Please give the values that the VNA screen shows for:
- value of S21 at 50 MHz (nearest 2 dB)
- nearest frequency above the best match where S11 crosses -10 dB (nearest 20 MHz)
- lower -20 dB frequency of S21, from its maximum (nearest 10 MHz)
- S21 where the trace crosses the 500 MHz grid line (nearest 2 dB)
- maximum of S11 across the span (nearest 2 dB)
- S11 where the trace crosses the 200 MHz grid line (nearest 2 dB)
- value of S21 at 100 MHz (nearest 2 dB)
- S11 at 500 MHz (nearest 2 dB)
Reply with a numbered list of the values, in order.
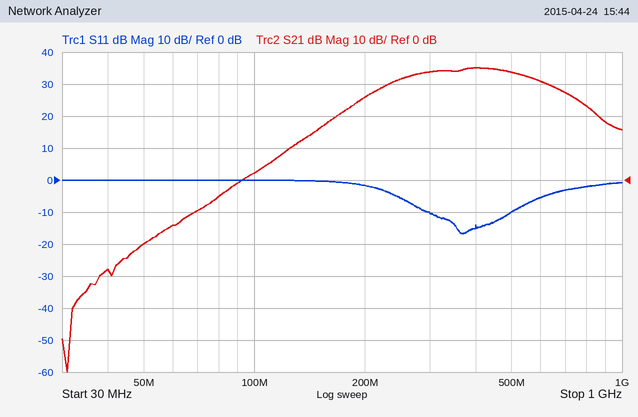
1. -20 dB
2. 500 MHz
3. 150 MHz
4. 34 dB
5. 0 dB
6. -2 dB
7. 2 dB
8. -10 dB
